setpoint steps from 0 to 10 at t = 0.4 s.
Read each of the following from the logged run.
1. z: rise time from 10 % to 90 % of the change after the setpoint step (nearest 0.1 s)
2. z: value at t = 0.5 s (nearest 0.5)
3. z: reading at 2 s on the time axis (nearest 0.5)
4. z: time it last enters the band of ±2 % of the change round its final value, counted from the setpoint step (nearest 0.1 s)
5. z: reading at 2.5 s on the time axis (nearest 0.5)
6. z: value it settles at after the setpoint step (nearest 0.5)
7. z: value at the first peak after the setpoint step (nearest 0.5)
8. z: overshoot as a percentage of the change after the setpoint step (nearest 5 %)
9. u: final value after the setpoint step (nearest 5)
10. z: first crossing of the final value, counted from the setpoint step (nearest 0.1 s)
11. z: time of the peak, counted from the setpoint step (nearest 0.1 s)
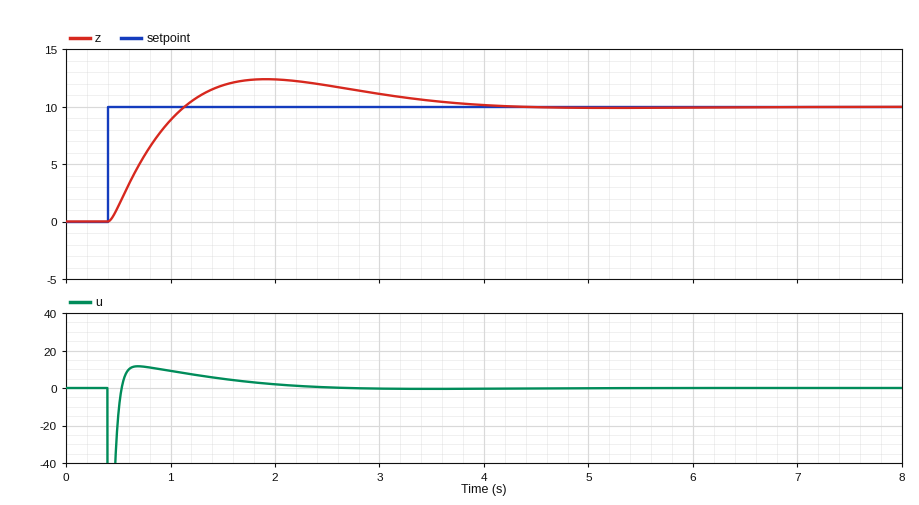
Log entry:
0.5 s
1.5
12.5
3.5 s
12.0
10.0
12.5
25 %
0
0.7 s
1.5 s
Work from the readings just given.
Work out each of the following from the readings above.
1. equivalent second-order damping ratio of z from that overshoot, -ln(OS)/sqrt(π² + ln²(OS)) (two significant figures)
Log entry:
0.40
